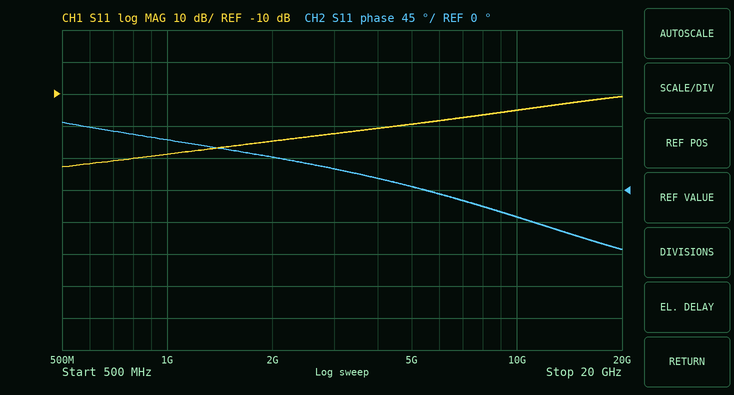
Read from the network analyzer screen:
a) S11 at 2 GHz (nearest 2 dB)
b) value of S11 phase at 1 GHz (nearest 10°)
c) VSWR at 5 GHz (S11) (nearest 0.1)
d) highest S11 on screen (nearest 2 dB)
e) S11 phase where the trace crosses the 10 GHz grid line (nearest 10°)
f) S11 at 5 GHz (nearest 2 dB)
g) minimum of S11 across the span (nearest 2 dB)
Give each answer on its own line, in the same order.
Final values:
-24 dB
70°
1.2
-10 dB
-40°
-20 dB
-32 dB
